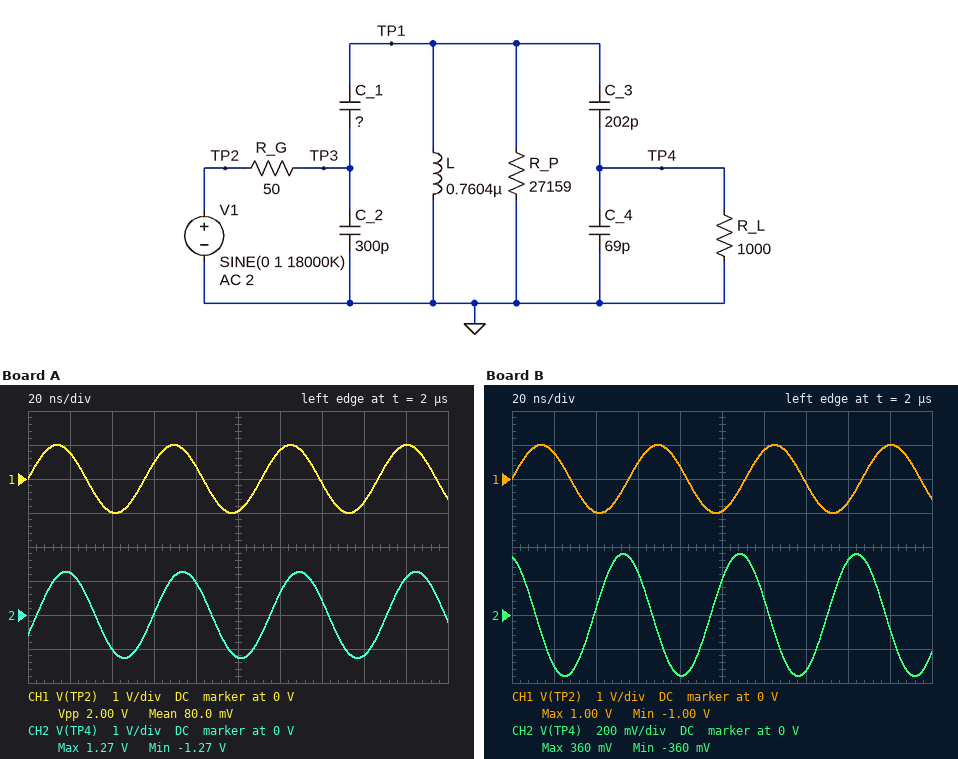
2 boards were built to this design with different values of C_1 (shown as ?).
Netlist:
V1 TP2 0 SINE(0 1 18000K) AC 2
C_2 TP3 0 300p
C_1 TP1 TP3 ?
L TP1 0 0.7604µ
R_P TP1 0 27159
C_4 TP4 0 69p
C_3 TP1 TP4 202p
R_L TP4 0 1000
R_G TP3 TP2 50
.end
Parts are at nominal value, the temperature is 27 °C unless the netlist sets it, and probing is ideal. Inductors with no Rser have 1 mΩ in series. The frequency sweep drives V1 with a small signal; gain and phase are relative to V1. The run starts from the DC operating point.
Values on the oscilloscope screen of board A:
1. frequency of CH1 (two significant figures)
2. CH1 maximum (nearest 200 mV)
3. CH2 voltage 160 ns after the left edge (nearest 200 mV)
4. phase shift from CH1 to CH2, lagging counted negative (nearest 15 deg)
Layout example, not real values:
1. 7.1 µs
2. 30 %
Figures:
1. 18 MHz
2. 1.0 V
3. -1.2 V
4. -30 deg
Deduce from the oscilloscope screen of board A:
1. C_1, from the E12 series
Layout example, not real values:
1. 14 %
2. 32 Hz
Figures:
1. 82 pF
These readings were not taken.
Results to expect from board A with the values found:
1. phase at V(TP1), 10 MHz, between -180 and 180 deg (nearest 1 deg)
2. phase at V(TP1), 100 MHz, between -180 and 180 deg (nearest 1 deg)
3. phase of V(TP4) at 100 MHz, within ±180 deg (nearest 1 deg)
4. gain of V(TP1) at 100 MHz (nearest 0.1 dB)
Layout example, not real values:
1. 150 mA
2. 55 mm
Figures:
1. 125 deg
2. -84 deg
3. -84 deg
4. -24.4 dB
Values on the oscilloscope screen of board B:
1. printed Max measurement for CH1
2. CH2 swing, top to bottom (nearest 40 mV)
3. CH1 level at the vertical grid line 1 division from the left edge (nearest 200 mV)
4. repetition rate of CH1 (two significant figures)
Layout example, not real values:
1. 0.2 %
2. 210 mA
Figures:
1. 1.00 V
2. 720 mV
3. 800 mV
4. 18 MHz
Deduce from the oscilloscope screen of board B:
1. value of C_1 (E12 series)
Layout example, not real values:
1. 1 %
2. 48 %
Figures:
1. 27 pF
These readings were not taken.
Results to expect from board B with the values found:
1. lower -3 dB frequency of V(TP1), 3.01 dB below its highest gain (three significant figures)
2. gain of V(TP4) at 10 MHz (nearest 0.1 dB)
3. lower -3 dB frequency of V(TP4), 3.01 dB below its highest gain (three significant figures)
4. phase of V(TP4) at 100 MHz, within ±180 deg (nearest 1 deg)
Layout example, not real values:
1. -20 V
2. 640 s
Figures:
1. 20.1 MHz
2. -25.2 dB
3. 20.1 MHz
4. -83 deg
